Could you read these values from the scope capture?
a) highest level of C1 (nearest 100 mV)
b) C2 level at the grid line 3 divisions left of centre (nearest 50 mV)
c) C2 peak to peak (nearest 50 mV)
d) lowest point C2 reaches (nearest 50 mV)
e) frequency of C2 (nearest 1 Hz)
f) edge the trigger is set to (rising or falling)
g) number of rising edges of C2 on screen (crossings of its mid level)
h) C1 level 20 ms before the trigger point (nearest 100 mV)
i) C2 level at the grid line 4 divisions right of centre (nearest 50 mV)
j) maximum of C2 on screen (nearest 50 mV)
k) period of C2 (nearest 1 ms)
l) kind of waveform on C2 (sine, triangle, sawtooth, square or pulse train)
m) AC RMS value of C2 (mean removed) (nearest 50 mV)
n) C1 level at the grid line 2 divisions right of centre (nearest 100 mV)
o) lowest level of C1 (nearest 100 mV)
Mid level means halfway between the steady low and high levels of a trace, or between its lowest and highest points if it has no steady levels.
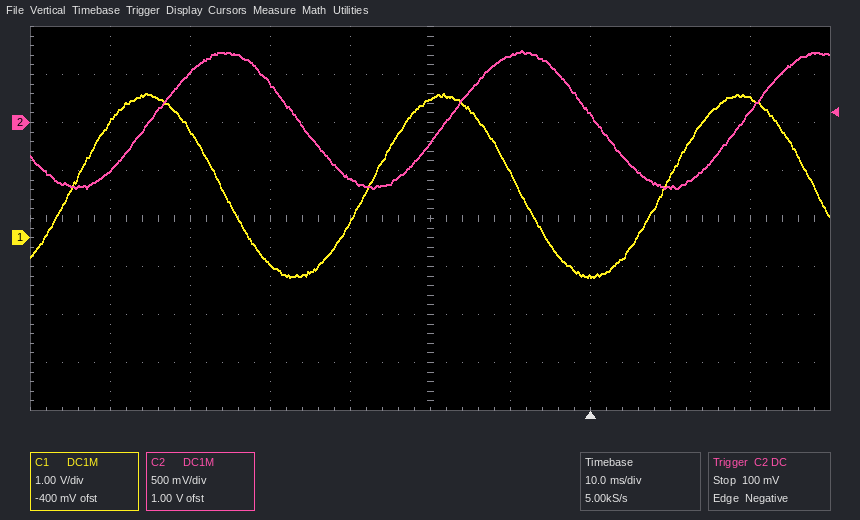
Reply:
3.0 V
500 mV
1.45 V
-700 mV
27 Hz
falling
3
2.9 V
100 mV
750 mV
37 ms
sine
500 mV
-800 mV
-800 mV
